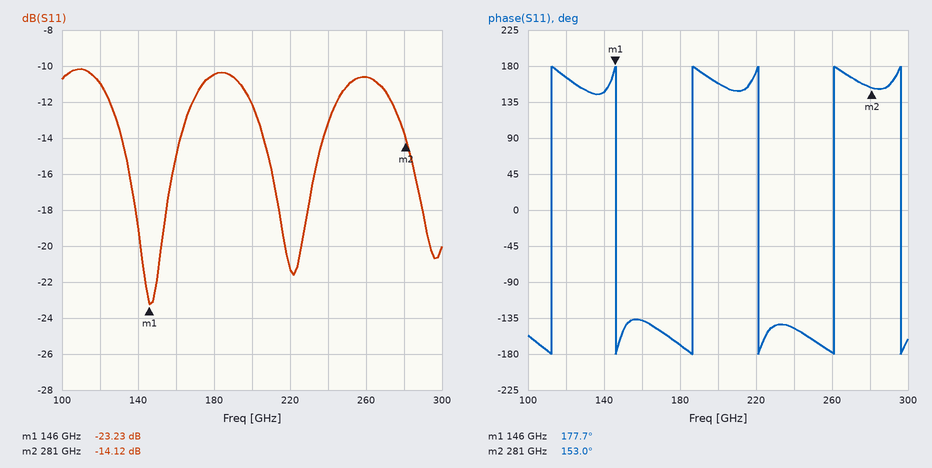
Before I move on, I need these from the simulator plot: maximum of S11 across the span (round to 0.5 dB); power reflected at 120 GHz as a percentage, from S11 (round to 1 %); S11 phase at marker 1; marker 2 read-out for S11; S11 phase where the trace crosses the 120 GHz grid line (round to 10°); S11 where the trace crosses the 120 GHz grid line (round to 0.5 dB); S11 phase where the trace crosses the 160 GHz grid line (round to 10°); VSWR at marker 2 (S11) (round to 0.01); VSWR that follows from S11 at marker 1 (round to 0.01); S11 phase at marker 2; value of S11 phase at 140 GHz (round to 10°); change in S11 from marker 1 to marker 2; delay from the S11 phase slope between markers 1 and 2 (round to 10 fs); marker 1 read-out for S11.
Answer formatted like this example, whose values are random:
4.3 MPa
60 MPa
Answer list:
-10.0 dB
8 %
177.7°
-14.12 dB
170°
-11.0 dB
-140°
1.49
1.15
153.0°
150°
9.11 dB
510 fs
-23.23 dB
